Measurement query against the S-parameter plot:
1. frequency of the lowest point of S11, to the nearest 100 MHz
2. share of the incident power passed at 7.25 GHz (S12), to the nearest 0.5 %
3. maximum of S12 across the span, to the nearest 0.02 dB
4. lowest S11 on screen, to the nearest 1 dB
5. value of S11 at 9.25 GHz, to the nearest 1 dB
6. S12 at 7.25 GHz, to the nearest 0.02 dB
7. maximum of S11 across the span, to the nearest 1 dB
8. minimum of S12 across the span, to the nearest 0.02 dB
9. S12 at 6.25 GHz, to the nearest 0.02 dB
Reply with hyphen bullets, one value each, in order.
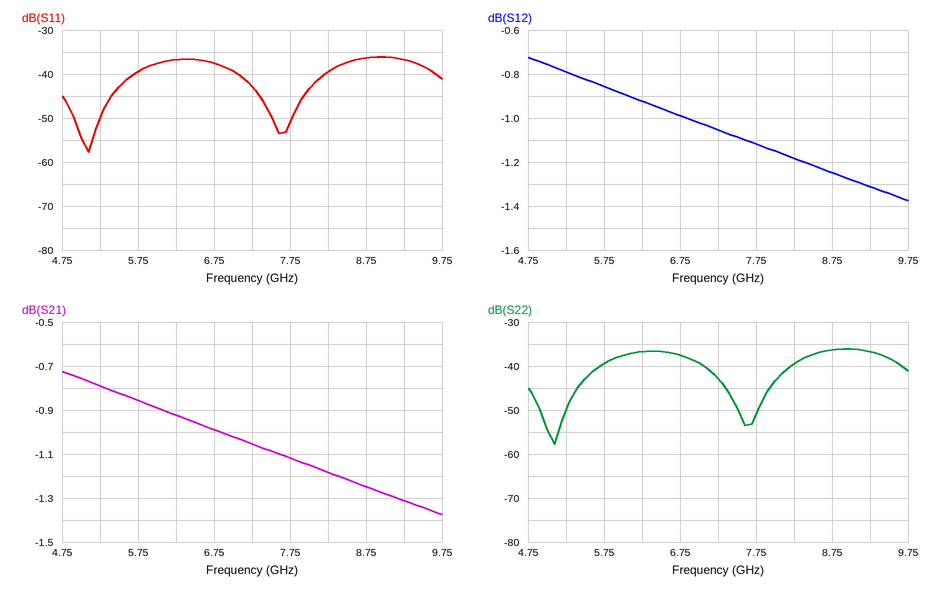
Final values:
- 5.1 GHz
- 78.5 %
- -0.72 dB
- -58 dB
- -37 dB
- -1.06 dB
- -36 dB
- -1.38 dB
- -0.92 dB
